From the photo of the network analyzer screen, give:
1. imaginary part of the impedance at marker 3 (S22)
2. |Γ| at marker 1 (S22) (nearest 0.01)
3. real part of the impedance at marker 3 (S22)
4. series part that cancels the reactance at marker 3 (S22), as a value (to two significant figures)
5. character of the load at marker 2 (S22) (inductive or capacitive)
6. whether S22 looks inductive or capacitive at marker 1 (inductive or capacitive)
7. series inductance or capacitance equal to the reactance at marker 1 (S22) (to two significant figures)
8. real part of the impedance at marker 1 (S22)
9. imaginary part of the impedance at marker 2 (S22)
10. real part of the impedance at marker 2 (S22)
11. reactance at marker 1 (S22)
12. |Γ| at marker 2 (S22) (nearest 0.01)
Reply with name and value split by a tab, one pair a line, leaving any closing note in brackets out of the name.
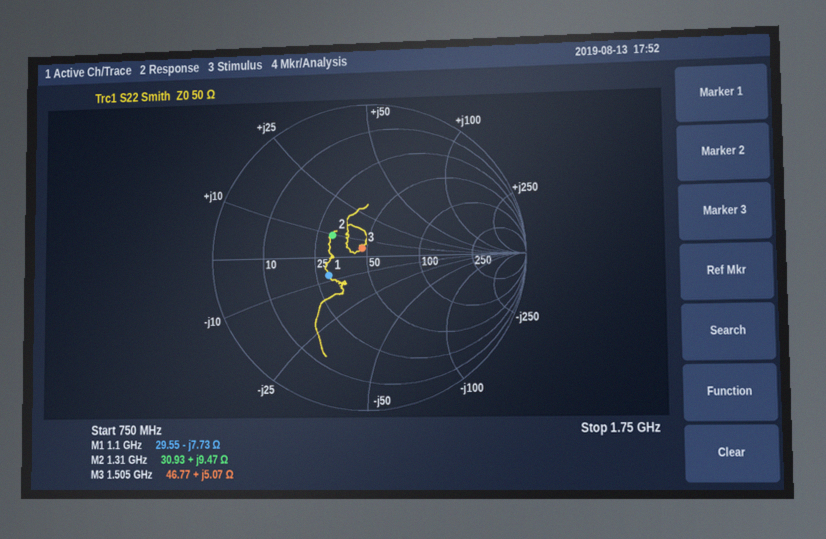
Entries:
imaginary part of the impedance at marker 3	+5.07 Ω
|Γ| at marker 1 (S22)	0.27
real part of the impedance at marker 3	46.77 Ω
series part that cancels the reactance at marker 3 (S22), as a value	21 pF
character of the load at marker 2 (S22)	inductive
whether S22 looks inductive or capacitive at marker 1	capacitive
series inductance or capacitance equal to the reactance at marker 1 (S22)	19 pF
real part of the impedance at marker 1	29.55 Ω
imaginary part of the impedance at marker 2	+9.47 Ω
real part of the impedance at marker 2	30.93 Ω
reactance at marker 1	-7.73 Ω
|Γ| at marker 2 (S22)	0.26
